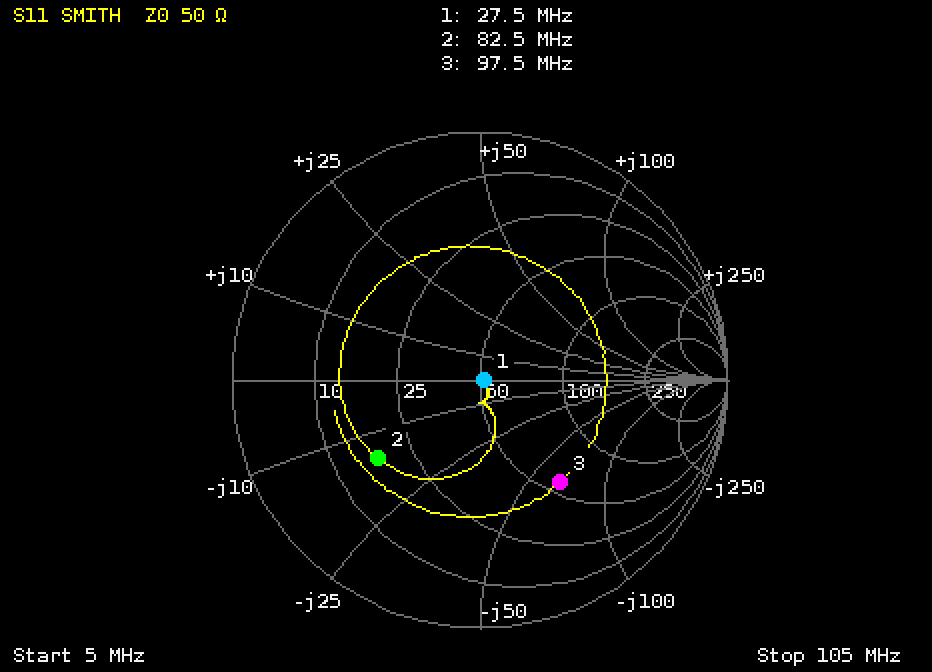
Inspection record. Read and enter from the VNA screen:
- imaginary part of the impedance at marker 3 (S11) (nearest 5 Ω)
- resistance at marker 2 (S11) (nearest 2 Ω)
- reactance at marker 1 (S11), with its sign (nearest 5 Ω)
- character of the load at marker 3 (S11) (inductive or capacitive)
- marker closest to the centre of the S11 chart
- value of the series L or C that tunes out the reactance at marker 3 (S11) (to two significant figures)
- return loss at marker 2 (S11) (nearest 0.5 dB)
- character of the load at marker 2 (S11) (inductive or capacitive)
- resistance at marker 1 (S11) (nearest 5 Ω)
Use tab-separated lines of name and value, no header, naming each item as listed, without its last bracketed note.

imaginary part of the impedance at marker 3 (S11)	-65 Ω
resistance at marker 2 (S11)	18 Ω
reactance at marker 1 (S11), with its sign	0 Ω
character of the load at marker 3 (S11)	capacitive
marker closest to the centre of the S11 chart	marker 1
value of the series L or C that tunes out the reactance at marker 3 (S11)	110 nH
return loss at marker 2 (S11)	5.5 dB
character of the load at marker 2 (S11)	capacitive
resistance at marker 1 (S11)	50 Ω
